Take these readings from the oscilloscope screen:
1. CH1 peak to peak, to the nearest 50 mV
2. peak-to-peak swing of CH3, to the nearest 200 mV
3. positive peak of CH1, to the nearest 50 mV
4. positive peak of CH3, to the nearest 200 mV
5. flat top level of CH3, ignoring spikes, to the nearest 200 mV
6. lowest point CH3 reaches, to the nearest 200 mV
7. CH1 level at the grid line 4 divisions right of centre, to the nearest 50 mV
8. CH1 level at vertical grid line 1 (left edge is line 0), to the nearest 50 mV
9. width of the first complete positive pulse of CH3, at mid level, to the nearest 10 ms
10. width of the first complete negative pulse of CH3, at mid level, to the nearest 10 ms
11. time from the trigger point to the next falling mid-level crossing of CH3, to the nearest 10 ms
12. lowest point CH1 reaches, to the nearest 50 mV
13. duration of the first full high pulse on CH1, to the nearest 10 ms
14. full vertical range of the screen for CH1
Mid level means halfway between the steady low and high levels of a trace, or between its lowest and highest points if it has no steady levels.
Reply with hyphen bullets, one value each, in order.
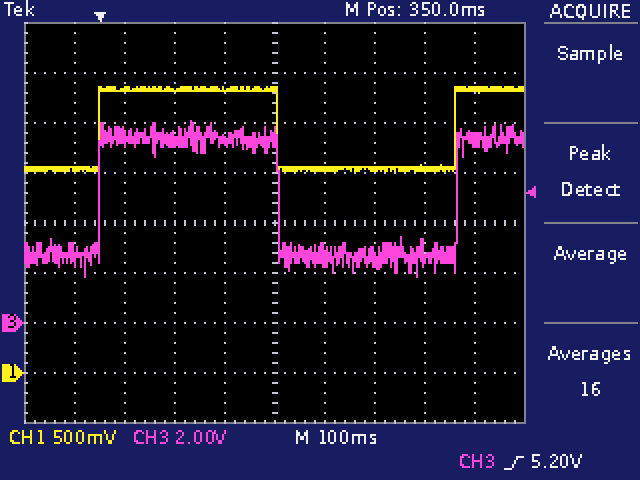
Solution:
- 850 mV
- 6.2 V
- 2.85 V
- 8.0 V
- 7.4 V
- 1.8 V
- 2.85 V
- 2.05 V
- 360 ms
- 360 ms
- 360 ms
- 2.00 V
- 360 ms
- 4 V
